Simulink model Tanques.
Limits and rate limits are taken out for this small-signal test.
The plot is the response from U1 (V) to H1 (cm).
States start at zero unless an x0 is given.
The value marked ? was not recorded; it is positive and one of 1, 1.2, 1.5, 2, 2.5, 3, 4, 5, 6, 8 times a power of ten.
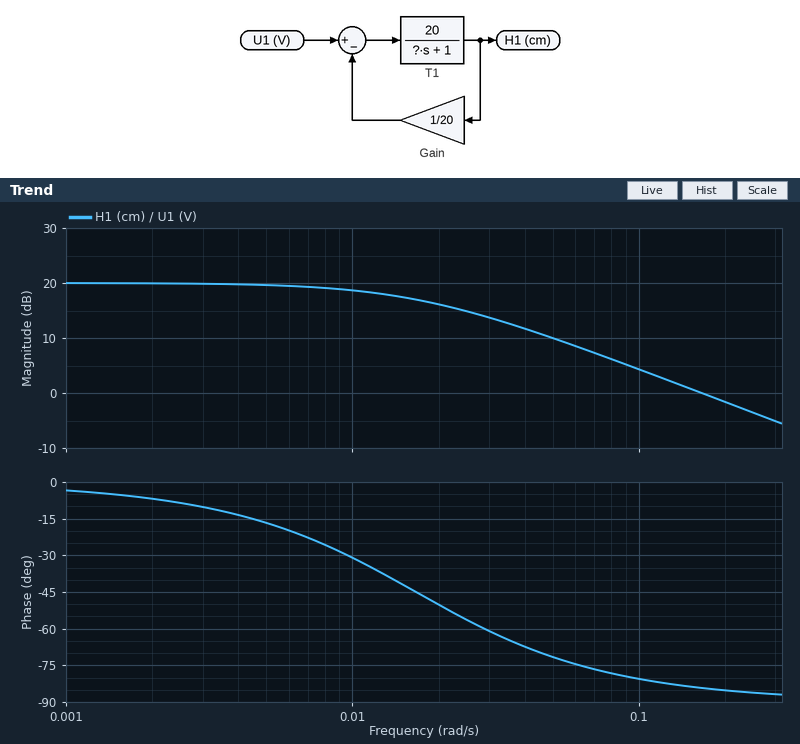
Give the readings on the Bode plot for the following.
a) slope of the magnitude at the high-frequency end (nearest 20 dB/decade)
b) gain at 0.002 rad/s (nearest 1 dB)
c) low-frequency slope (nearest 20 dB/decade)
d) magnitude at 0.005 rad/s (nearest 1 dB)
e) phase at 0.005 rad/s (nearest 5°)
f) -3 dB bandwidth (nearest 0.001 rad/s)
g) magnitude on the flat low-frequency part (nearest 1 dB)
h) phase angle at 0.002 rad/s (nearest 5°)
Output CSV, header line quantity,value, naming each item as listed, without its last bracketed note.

quantity,value
slope of the magnitude at the high-frequency end,-20 dB/decade
gain at 0.002 rad/s,20 dB
low-frequency slope,0 dB/decade
magnitude at 0.005 rad/s,20 dB
phase at 0.005 rad/s,-15°
-3 dB bandwidth,0.017 rad/s
magnitude on the flat low-frequency part,20 dB
phase angle at 0.002 rad/s,-5°
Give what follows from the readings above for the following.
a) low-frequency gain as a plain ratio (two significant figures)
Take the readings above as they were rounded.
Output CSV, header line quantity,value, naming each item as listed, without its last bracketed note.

quantity,value
low-frequency gain as a plain ratio,10
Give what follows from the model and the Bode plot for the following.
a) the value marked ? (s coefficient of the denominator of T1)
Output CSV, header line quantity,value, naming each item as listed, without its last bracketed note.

quantity,value
the value marked ?,120
